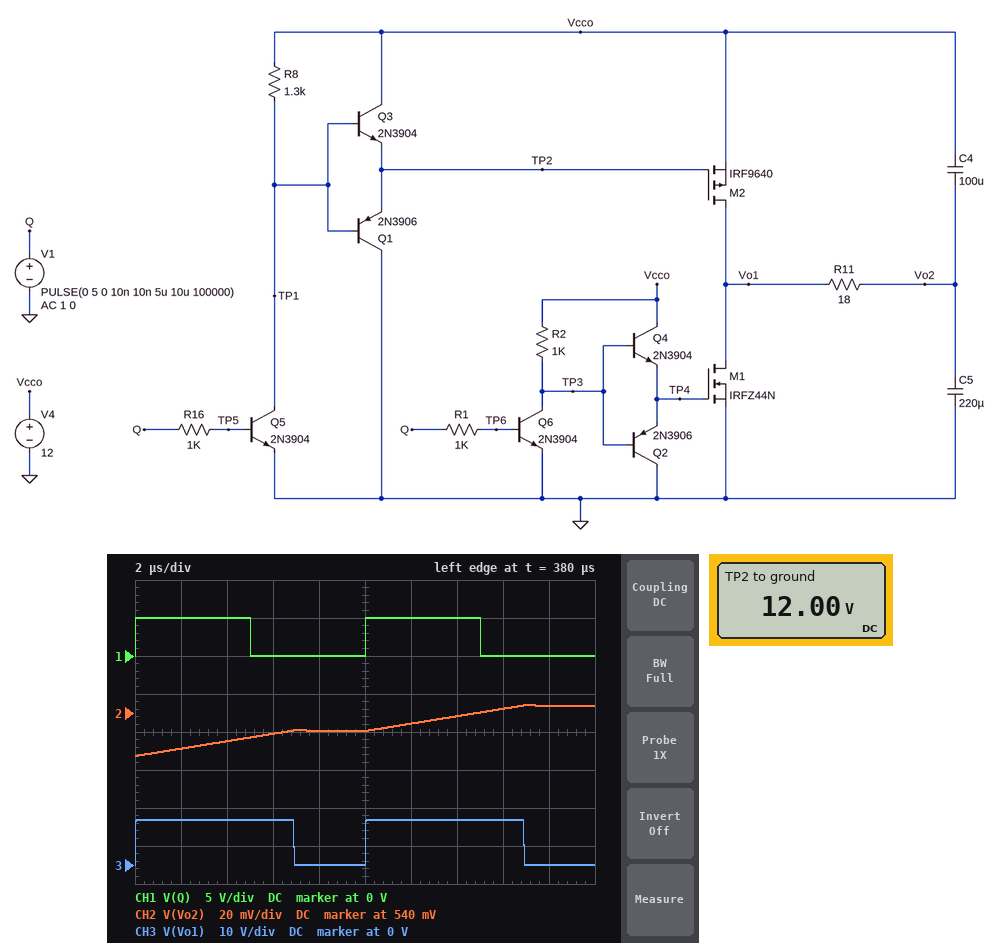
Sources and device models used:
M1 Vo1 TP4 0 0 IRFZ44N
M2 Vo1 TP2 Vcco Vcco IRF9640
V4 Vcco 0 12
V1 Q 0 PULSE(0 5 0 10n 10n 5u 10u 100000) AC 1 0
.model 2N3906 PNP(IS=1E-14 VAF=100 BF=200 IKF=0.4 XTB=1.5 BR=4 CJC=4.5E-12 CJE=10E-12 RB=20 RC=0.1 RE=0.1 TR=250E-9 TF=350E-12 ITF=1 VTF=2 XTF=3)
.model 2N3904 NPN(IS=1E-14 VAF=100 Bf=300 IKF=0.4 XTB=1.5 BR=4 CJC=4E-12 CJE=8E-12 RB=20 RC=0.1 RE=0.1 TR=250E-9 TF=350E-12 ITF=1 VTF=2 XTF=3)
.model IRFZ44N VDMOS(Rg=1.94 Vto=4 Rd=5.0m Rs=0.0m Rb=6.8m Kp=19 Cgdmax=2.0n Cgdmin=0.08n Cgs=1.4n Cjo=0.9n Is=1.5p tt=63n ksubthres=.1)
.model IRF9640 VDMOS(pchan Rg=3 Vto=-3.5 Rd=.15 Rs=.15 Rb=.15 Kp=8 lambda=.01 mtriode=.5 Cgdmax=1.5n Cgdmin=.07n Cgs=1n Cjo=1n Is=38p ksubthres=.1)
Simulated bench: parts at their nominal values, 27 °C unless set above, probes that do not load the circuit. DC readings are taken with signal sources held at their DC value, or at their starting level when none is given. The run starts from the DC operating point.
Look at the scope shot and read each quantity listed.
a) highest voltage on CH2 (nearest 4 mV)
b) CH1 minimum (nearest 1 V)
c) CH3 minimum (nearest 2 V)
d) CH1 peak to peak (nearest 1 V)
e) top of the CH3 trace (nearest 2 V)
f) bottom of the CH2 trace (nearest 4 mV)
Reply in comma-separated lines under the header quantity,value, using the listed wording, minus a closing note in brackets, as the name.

quantity,value
highest voltage on CH2,544 mV
CH1 minimum,0 V
CH3 minimum,0 V
CH1 peak to peak,5 V
top of the CH3 trace,12 V
bottom of the CH2 trace,516 mV
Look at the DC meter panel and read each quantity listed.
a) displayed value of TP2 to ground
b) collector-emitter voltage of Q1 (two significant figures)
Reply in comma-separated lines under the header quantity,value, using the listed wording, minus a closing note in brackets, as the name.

quantity,value
displayed value of TP2 to ground,12.00 V
collector-emitter voltage of Q1,-12 V
